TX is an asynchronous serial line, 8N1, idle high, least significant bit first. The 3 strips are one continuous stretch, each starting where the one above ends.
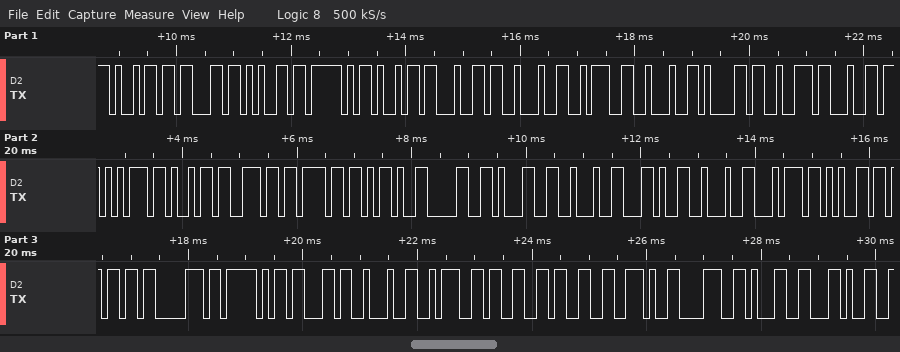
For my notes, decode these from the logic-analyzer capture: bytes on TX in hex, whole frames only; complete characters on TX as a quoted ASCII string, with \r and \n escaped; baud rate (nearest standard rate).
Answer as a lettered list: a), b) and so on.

a) 69 63 65 5F 69 64 22 3A 22 61 72 64 75 69 6E 6F 2D 30 31 22 2C 22 74 65 6D 70 5F 63 22 3A 33 33 2E 38 31 2C
b) "ice_id\":\"arduino-01\",\"temp_c\":33.81,"
c) 9600 baud
